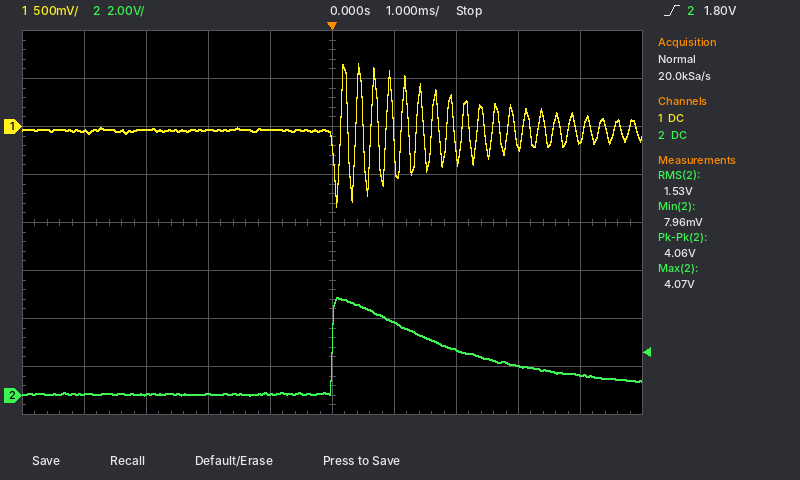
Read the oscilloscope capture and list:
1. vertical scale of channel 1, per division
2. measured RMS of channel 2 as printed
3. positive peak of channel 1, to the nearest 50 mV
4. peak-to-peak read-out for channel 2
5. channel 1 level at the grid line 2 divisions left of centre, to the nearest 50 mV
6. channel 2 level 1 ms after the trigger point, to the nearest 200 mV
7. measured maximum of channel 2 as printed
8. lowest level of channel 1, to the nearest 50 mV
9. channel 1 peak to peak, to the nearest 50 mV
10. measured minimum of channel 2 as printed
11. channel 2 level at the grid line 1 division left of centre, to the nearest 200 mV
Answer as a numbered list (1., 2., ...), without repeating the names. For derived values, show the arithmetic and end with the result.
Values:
1. 500 mV
2. 1.53 V
3. 650 mV
4. 4.06 V
5. -50 mV
6. 3.0 V
7. 4.07 V
8. -850 mV
9. 650 mV − (-850 mV) = 1.50 V
10. 7.96 mV
11. 0.0 V
